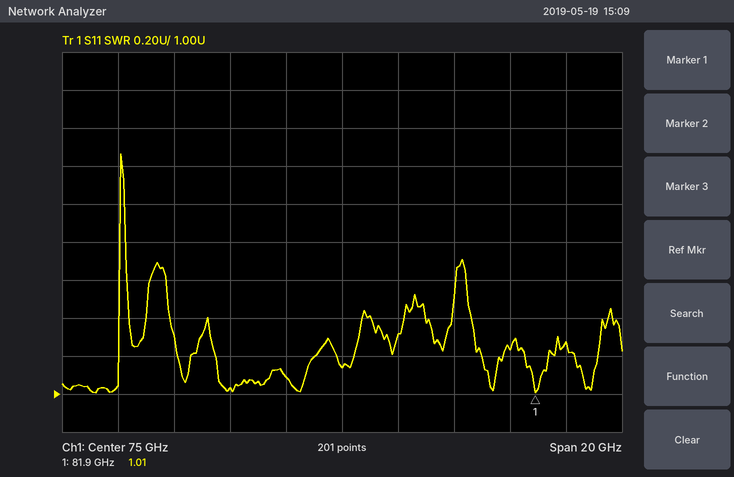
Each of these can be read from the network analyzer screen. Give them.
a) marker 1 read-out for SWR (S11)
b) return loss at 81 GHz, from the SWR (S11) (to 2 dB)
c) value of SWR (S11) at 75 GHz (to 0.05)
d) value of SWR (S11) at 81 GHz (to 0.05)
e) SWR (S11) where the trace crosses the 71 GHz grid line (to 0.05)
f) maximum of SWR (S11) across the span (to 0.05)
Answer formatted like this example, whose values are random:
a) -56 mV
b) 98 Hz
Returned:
a) 1.01
b) 20 dB
c) 1.15
d) 1.25
e) 1.05
f) 2.25
